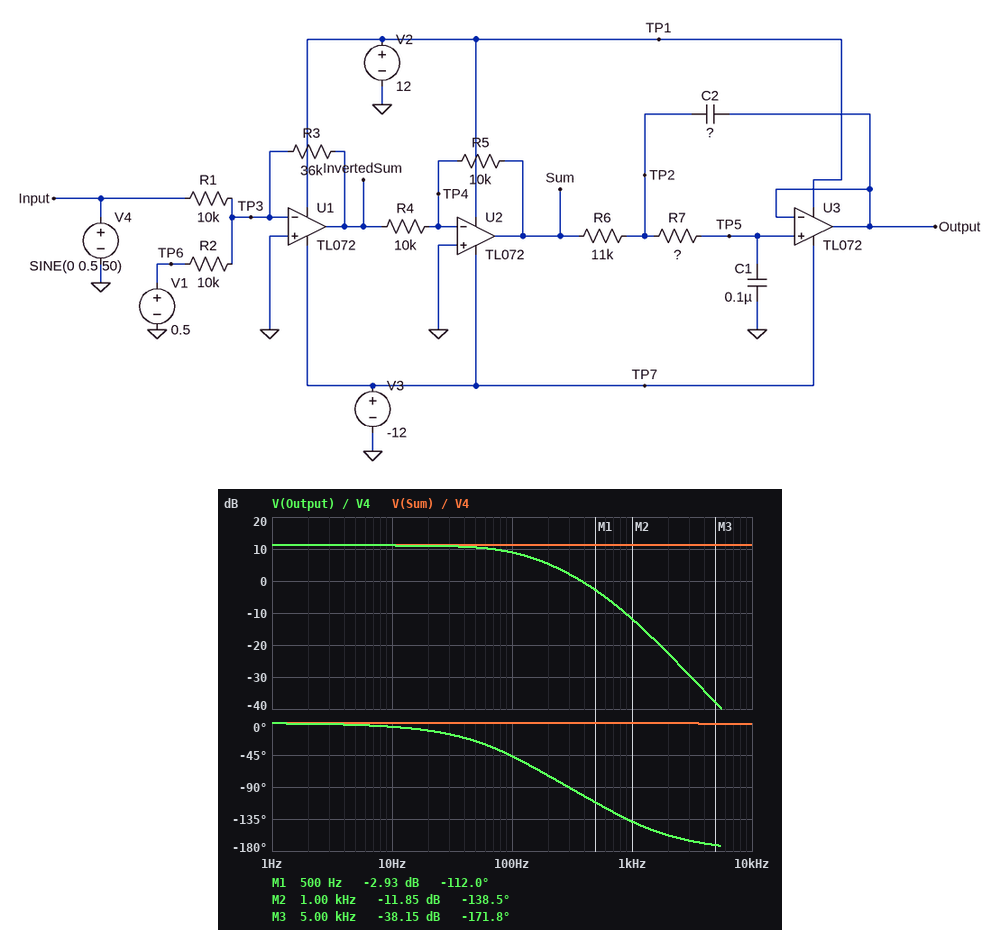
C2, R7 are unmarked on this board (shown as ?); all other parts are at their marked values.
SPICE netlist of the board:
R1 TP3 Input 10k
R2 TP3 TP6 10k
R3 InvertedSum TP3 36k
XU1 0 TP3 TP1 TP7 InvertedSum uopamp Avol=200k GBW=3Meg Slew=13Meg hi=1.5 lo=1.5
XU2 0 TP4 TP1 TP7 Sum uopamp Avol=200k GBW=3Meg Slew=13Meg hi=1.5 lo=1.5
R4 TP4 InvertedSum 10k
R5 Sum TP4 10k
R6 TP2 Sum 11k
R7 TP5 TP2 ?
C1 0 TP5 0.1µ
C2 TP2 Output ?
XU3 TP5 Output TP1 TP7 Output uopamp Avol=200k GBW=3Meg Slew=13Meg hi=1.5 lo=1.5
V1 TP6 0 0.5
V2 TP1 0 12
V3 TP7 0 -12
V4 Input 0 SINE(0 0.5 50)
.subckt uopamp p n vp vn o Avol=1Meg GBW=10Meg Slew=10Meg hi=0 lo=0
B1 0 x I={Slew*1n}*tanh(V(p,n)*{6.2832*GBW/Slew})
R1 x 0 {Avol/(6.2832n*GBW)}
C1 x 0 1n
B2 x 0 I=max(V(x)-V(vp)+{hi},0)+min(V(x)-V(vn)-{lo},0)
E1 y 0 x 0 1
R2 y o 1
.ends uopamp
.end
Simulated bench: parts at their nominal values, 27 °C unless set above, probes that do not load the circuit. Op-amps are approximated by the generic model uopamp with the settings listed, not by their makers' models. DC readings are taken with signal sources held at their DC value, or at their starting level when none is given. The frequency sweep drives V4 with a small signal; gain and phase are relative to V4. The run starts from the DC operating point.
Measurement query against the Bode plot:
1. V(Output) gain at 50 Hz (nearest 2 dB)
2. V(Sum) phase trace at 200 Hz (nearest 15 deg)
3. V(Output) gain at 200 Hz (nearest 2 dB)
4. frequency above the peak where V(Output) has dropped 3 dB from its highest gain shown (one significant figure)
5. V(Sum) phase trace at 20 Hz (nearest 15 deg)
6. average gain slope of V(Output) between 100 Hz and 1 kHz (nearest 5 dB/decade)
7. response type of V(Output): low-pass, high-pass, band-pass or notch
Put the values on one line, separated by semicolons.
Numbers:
10 dB; 0 deg; 6 dB; 100 Hz; 0 deg; -20 dB/decade; low-pass
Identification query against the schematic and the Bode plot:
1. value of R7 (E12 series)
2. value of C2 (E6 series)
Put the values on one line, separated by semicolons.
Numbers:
3.9 kΩ; 68 nF
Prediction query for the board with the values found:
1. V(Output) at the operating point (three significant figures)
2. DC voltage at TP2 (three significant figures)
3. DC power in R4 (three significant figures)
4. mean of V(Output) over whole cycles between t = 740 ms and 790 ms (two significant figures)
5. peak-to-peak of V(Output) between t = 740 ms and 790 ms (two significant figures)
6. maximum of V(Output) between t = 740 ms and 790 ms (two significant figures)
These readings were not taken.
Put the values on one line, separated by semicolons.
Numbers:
1.80 V; 1.80 V; 324 µW; 1.8 V; 3.3 V; 3.5 V
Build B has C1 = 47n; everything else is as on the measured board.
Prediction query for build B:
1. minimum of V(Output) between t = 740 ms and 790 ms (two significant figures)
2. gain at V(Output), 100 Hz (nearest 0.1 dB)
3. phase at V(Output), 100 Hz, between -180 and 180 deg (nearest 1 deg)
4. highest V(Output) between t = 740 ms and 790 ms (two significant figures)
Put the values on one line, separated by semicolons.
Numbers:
19 mV; 10.8 dB; -25 deg; 3.6 V
